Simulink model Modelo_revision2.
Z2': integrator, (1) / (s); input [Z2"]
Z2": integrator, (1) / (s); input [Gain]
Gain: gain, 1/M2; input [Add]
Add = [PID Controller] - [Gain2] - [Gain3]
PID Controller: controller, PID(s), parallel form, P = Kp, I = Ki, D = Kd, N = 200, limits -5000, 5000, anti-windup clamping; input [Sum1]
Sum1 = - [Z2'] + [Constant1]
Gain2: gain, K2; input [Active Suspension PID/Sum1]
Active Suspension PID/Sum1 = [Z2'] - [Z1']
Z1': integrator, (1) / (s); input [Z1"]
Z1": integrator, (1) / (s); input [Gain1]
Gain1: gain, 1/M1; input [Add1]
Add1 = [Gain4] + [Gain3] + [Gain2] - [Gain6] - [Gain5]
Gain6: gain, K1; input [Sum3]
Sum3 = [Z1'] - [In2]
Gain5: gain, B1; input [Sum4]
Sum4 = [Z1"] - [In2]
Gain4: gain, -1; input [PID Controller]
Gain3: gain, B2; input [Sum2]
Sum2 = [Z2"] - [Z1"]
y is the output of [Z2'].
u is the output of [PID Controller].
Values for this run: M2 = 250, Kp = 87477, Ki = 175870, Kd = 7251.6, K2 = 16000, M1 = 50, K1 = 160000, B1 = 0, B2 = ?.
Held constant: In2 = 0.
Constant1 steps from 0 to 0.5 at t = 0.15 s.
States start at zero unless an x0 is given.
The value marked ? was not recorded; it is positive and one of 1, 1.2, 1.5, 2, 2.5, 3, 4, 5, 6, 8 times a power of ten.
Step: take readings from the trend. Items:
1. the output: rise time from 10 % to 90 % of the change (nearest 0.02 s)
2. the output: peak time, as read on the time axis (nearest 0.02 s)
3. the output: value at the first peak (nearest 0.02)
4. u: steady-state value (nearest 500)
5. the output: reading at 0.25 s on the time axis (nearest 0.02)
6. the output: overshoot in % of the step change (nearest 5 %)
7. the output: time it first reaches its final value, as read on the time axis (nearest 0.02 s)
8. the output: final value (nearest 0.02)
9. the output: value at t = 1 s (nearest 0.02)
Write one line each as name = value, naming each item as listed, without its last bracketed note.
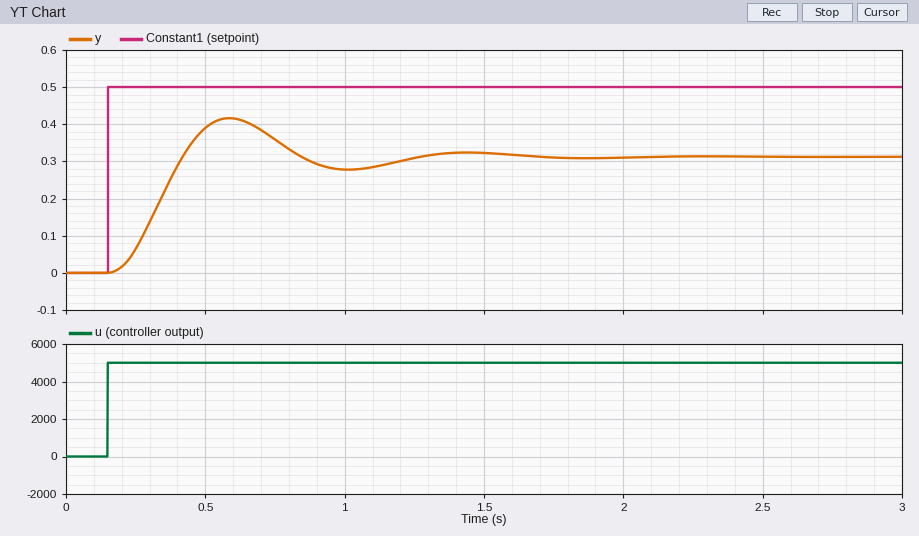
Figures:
the output: rise time from 10 % to 90 % of the change = 0.18 s
the output: peak time, as read on the time axis = 0.58 s
the output: value at the first peak = 0.42
u: steady-state value = 5000
the output: reading at 0.25 s on the time axis = 0.06
the output: overshoot in % of the step change = 35 %
the output: time it first reaches its final value, as read on the time axis = 0.42 s
the output: final value = 0.32
the output: value at t = 1 s = 0.28
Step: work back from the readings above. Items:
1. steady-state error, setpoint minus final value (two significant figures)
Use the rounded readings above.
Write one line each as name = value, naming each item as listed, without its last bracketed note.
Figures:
steady-state error, setpoint minus final value = 0.18
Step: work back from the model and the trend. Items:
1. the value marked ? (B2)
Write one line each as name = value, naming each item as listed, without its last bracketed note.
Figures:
the value marked ? = 1500
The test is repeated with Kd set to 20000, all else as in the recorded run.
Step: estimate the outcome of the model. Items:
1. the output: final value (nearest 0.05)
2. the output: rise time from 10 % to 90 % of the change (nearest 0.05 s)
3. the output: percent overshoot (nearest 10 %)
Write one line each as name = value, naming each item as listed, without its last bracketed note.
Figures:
the output: final value = 0.30
the output: rise time from 10 % to 90 % of the change = 0.20 s
the output: percent overshoot = 20 %
